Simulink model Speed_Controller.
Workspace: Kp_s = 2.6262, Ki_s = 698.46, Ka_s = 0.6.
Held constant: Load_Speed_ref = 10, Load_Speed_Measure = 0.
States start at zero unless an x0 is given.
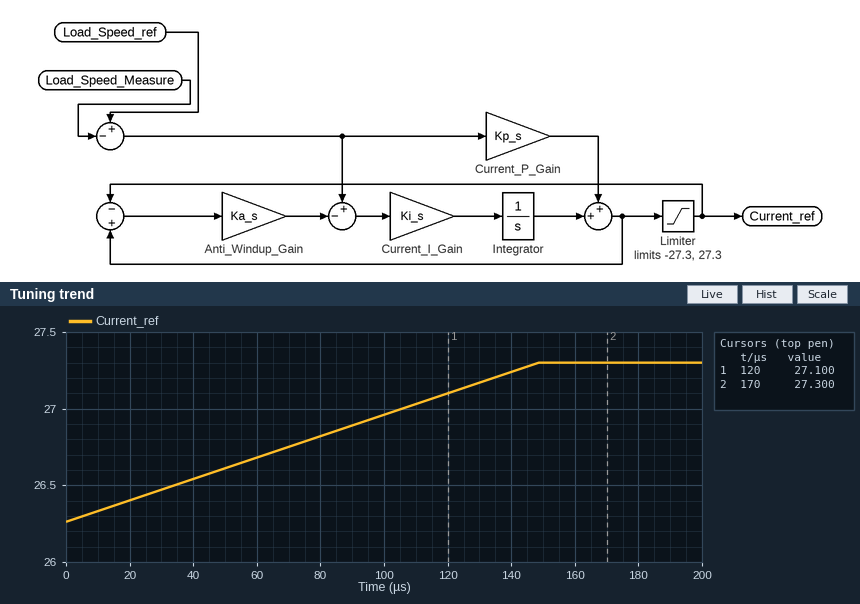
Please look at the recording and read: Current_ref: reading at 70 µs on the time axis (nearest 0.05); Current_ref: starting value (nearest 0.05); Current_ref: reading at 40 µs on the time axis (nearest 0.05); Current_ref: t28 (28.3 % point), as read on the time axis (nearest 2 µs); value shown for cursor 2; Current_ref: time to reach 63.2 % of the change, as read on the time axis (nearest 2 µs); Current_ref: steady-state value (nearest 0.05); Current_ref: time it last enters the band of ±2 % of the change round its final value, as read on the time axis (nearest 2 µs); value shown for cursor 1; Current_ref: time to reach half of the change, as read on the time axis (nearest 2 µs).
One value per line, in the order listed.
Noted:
26.75
26.25
26.55
42 µs
27.300
94 µs
27.30
146 µs
27.100
74 µs
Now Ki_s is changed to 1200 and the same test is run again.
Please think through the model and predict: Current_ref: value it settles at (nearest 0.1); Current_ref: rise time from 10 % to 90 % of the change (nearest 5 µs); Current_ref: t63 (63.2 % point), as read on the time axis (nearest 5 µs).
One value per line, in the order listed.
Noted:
27.3
70 µs
55 µs
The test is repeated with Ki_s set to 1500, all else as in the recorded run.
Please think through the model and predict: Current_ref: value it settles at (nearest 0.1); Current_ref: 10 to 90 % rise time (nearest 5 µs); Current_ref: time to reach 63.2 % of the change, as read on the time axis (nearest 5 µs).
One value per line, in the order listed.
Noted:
27.3
55 µs
45 µs
